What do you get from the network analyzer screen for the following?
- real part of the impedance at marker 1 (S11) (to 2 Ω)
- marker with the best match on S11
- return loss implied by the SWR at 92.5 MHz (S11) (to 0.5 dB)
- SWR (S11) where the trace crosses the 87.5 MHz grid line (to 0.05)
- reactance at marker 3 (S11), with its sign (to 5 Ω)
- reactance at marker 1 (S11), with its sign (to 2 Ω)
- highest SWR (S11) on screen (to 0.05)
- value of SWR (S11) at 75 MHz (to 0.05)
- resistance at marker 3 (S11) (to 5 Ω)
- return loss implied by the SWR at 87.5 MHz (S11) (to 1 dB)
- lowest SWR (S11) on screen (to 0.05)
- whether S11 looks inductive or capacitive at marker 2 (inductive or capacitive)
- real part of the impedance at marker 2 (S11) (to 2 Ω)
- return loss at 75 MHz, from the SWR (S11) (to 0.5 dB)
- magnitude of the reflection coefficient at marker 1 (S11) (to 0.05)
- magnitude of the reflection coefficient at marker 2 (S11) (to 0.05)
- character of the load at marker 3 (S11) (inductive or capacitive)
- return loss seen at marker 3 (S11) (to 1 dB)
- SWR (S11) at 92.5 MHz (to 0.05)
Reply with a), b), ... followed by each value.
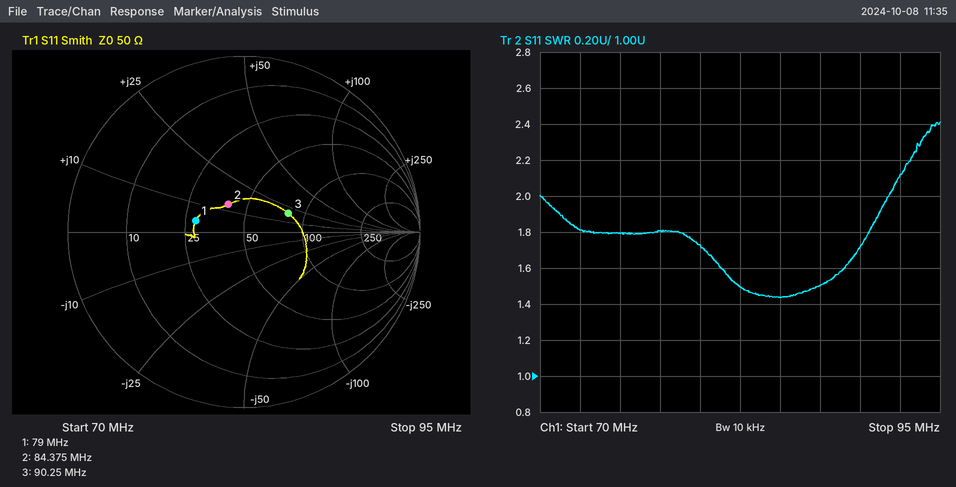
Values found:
a) 28 Ω
b) marker 2
c) 9.0 dB
d) 1.50
e) +20 Ω
f) +4 Ω
g) 2.40
h) 1.80
i) 80 Ω
j) 14 dB
k) 1.45
l) inductive
m) 40 Ω
n) 11.0 dB
o) 0.30
p) 0.20
q) inductive
r) 11 dB
s) 2.10
